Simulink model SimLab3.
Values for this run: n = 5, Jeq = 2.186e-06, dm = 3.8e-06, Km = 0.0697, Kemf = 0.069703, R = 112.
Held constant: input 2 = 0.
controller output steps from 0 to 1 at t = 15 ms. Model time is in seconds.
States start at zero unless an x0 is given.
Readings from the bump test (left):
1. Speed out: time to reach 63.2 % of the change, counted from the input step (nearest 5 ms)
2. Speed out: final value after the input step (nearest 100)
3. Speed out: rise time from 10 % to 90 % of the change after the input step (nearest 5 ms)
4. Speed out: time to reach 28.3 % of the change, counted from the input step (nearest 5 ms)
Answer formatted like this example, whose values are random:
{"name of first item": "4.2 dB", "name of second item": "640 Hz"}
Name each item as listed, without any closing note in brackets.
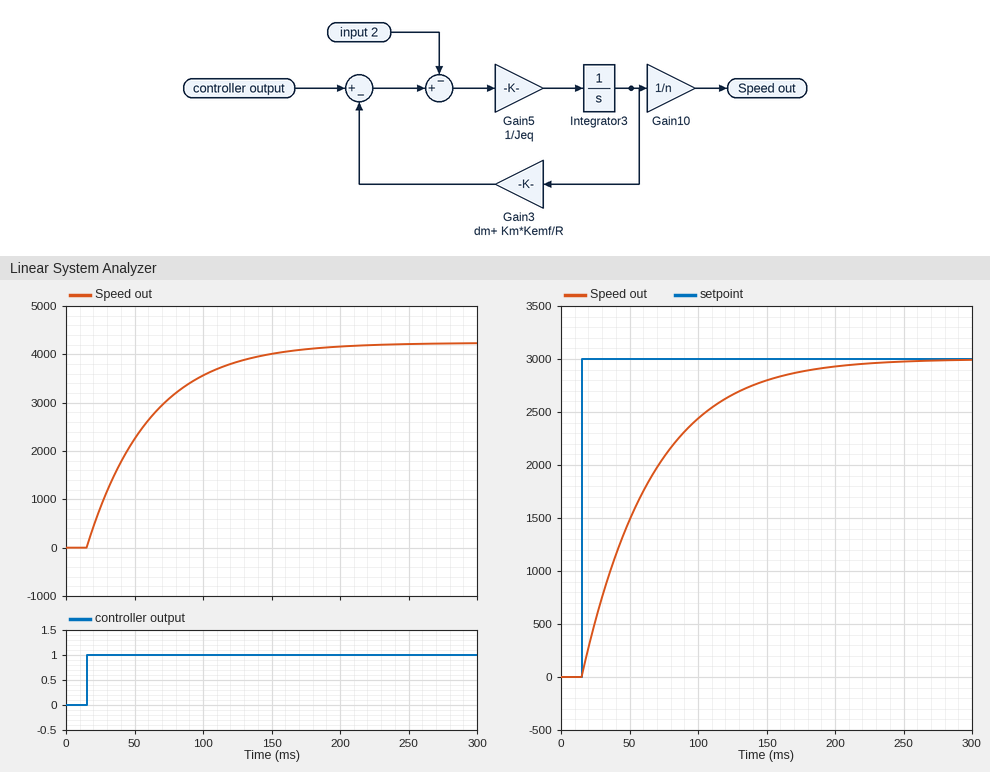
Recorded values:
{"Speed out: time to reach 63.2 % of the change, counted from the input step": "45 ms", "Speed out: final value after the input step": "4200", "Speed out: rise time from 10 % to 90 % of the change after the input step": "100 ms", "Speed out: time to reach 28.3 % of the change, counted from the input step": "15 ms"}
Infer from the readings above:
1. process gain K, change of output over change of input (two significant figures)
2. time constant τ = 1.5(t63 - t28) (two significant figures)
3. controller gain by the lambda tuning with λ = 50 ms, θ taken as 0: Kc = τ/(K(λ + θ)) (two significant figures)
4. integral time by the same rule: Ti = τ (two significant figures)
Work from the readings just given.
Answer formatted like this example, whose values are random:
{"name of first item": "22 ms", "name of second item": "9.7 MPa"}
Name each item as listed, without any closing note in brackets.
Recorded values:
{"process gain K, change of output over change of input": "4200", "time constant τ = 1.5(t63 - t28)": "45 ms", "controller gain by the lambda tuning with λ = 50 ms, θ taken as 0: Kc = τ/(K(λ + θ))": "0.00021", "integral time by the same rule: Ti = τ": "45 ms"}
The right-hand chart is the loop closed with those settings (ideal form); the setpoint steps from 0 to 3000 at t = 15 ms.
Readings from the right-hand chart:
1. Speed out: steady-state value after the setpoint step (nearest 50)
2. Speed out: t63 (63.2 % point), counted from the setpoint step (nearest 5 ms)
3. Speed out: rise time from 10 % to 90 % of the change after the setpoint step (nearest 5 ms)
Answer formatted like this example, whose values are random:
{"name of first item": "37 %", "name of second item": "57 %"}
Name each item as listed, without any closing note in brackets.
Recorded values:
{"Speed out: steady-state value after the setpoint step": "3000", "Speed out: t63 (63.2 % point), counted from the setpoint step": "50 ms", "Speed out: rise time from 10 % to 90 % of the change after the setpoint step": "110 ms"}
